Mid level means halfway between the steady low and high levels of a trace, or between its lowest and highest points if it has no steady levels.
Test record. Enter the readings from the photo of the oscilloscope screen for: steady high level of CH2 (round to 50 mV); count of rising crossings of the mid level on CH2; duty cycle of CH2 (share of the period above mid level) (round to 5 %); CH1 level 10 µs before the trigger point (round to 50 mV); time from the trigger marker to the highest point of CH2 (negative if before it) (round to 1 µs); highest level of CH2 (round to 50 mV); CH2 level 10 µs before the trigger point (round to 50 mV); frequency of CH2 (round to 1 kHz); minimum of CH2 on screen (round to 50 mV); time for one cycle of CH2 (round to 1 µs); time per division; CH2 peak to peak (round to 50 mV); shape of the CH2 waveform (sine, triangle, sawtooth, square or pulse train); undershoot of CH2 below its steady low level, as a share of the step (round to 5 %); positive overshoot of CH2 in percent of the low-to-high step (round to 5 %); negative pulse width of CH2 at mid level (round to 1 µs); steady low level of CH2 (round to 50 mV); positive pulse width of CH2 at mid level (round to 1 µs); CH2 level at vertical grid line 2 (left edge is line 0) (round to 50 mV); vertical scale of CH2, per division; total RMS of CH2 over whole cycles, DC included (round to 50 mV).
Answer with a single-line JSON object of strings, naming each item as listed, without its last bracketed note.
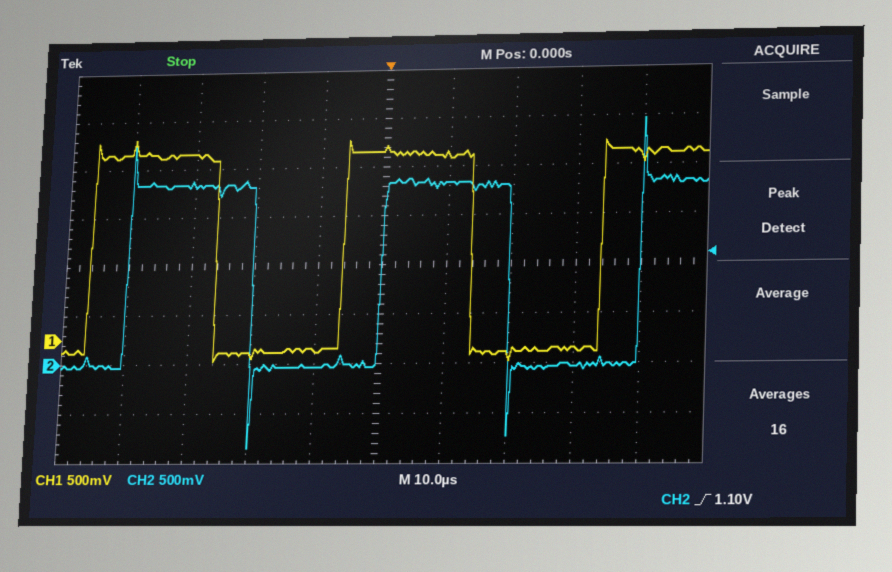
{"steady high level of CH2": "1.85 V", "count of rising crossings of the mid level on CH2": "3", "duty cycle of CH2 (share of the period above mid level)": "50 %", "CH1 level 10 µs before the trigger point": "-100 mV", "time from the trigger marker to the highest point of CH2 (negative if before it)": "+40 µs", "highest level of CH2": "2.45 V", "CH2 level 10 µs before the trigger point": "-50 mV", "frequency of CH2": "25 kHz", "minimum of CH2 on screen": "-850 mV", "time for one cycle of CH2": "40 µs", "time per division": "10 µs", "CH2 peak to peak": "3.30 V", "shape of the CH2 waveform": "square", "undershoot of CH2 below its steady low level, as a share of the step": "45 %", "positive overshoot of CH2 in percent of the low-to-high step": "35 %", "negative pulse width of CH2 at mid level": "20 µs", "steady low level of CH2": "-50 mV", "positive pulse width of CH2 at mid level": "20 µs", "CH2 level at vertical grid line 2 (left edge is line 0)": "1.85 V", "vertical scale of CH2, per division": "500 mV", "total RMS of CH2 over whole cycles, DC included": "1.30 V"}
